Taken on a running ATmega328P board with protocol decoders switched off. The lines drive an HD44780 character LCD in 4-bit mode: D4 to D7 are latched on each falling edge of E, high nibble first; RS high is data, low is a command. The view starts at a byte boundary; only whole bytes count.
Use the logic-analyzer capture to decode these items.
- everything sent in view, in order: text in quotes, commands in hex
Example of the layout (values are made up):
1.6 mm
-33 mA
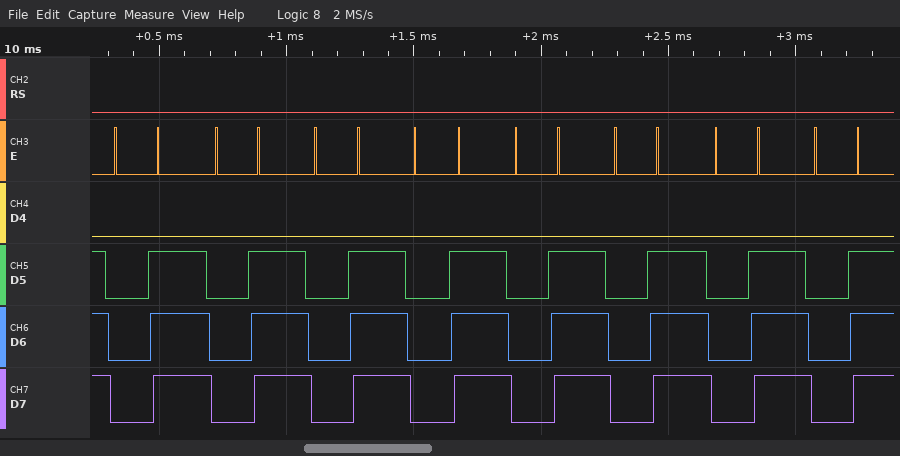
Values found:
0x0E 0x0E 0x0E 0x0E 0x0E 0x0E 0x0E 0x0E
